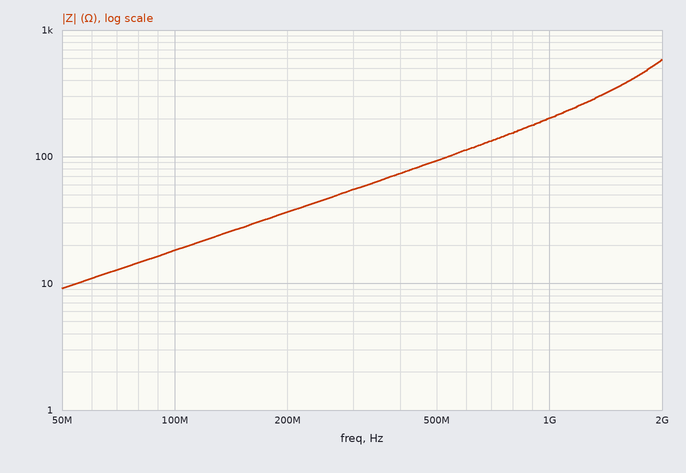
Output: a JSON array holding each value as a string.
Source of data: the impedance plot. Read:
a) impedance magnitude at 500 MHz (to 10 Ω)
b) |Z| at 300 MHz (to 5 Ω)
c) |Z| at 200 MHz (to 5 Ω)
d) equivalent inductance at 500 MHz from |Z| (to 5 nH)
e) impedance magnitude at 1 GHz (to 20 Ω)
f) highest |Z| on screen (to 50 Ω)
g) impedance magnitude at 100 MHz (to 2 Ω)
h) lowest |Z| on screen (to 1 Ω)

["90 Ω", "55 Ω", "35 Ω", "30 nH", "200 Ω", "600 Ω", "18 Ω", "9 Ω"]
